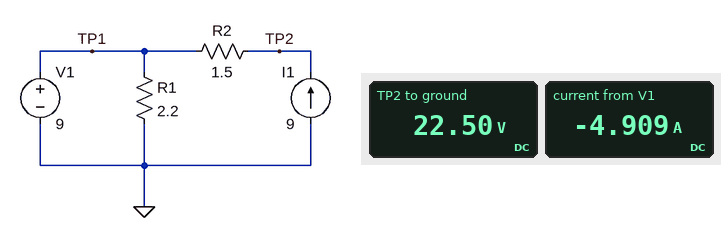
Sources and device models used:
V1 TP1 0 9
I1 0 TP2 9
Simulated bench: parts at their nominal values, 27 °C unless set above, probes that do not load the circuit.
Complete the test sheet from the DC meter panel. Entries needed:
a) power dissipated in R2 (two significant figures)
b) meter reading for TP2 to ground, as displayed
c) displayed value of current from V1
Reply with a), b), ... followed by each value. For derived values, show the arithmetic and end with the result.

a) (22.5 V - 9 V)^2 / 1.5 Ω = 120 W
b) 22.50 V
c) -4.909 A
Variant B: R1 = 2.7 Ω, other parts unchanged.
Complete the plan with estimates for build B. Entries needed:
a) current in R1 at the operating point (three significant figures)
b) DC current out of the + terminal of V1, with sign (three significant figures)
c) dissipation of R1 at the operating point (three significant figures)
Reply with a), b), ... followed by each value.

a) 3.33 A
b) -5.67 A
c) 30.0 W
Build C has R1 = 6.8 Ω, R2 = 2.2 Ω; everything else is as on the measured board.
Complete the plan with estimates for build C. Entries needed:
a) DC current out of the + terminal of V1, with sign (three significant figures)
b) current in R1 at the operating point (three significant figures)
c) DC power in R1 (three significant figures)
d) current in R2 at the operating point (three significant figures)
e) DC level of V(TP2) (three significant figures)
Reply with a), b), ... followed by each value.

a) -7.68 A
b) 1.32 A
c) 11.9 W
d) 9.00 A
e) 28.8 V
